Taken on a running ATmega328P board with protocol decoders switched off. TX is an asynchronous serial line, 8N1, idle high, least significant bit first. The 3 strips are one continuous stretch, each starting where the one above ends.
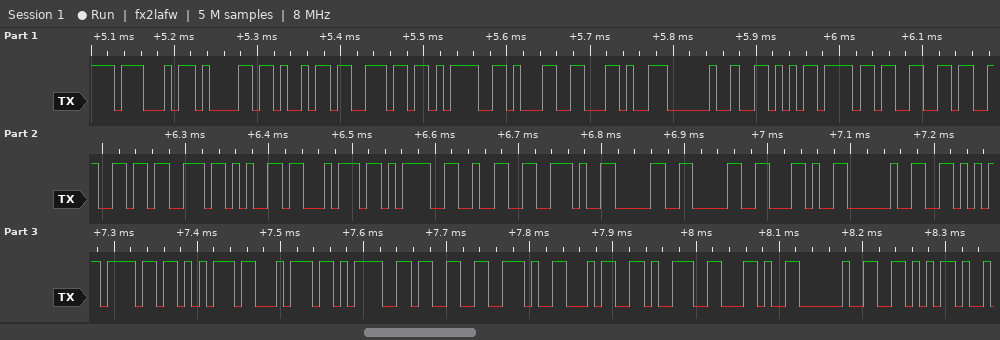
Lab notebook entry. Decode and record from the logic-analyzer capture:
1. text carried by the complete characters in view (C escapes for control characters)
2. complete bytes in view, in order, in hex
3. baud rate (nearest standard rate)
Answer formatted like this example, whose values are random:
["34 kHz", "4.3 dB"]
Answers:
["\"Gain=1, Voffset=2.00, Vout=3.49, V\"", "47 61 69 6E 3D 31 2C 20 56 6F 66 66 73 65 74 3D 32 2E 30 30 2C 20 56 6F 75 74 3D 33 2E 34 39 2C 20 56", "115200 baud"]
